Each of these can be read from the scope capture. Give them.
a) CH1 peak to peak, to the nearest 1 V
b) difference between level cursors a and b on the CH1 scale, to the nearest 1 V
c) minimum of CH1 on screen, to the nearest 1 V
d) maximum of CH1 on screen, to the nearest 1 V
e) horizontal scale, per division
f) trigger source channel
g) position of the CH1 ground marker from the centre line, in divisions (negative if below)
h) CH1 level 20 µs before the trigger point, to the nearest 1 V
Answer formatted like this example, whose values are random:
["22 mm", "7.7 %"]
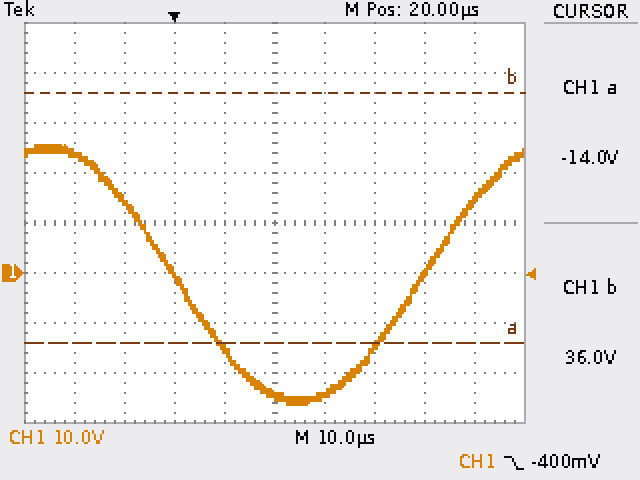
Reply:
["52 V", "50 V", "-26 V", "26 V", "10 µs", "CH1", "-1.0 div", "24 V"]
